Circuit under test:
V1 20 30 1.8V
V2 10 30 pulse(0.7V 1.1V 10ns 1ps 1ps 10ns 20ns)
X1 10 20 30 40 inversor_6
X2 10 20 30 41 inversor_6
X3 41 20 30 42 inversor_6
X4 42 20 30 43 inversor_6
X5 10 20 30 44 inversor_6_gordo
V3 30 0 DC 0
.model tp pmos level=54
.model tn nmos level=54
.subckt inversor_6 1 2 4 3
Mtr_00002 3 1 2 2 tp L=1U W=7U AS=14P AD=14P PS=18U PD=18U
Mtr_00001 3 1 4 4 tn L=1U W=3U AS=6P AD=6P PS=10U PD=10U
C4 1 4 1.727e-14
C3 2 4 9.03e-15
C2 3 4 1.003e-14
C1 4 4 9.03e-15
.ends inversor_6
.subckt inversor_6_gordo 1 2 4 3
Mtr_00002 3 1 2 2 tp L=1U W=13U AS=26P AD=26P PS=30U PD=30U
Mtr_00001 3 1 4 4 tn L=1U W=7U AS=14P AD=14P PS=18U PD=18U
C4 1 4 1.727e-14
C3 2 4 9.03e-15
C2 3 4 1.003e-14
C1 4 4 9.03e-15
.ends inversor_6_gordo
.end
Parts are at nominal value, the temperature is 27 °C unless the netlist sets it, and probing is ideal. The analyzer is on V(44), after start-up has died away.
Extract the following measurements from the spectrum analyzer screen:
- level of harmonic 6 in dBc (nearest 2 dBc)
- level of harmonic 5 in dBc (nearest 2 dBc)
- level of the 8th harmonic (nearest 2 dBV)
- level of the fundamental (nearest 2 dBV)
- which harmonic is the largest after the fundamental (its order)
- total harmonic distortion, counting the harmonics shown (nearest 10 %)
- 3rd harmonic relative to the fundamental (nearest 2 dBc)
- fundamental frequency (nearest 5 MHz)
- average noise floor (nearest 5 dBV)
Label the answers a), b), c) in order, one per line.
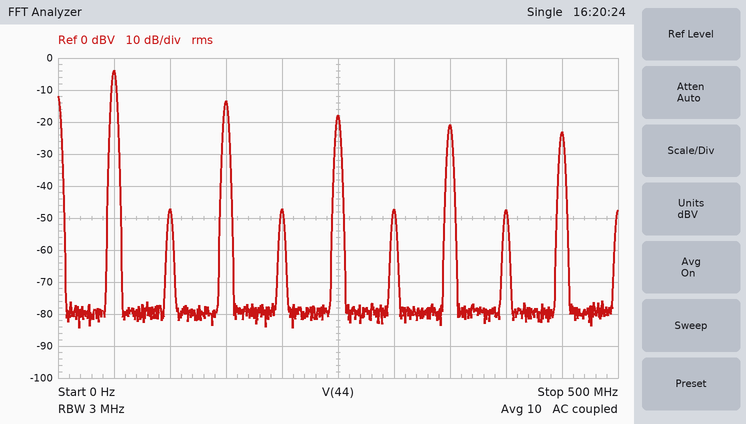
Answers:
a) -44 dBc
b) -14 dBc
c) -48 dBV
d) -4 dBV
e) 3
f) 40 %
g) -10 dBc
h) 50 MHz
i) -80 dBV
